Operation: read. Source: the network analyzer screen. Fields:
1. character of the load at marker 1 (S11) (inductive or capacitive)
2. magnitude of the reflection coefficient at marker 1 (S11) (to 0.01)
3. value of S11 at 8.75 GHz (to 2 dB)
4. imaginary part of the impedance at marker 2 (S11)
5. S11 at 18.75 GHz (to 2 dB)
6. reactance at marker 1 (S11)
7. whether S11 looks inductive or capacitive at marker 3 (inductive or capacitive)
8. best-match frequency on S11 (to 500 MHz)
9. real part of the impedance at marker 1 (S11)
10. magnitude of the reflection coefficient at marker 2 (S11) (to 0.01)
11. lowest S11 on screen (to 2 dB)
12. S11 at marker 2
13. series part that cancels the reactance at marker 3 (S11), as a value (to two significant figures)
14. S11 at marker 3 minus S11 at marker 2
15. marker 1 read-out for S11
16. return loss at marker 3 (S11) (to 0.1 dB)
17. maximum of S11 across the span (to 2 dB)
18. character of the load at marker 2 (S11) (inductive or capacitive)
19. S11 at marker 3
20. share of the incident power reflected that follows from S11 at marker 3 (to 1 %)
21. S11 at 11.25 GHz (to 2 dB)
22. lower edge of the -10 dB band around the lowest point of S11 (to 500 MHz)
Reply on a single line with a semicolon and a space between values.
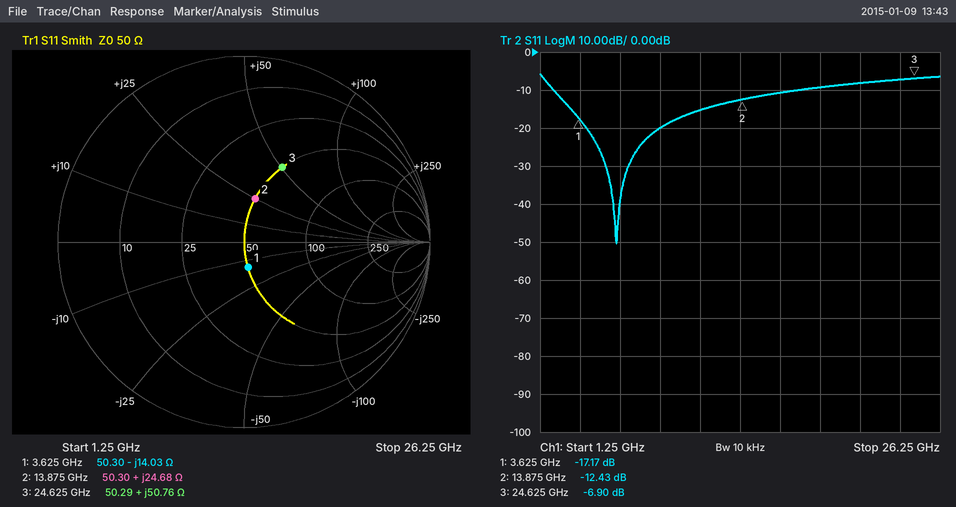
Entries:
capacitive; 0.14; -20 dB; +24.68 Ω; -10 dB; -14.03 Ω; inductive; 6.0 GHz; 50.30 Ω; 0.24; -50 dB; -12.43 dB; 130 fF; 5.53 dB; -17.17 dB; 6.9 dB; -6 dB; inductive; -6.90 dB; 20 %; -16 dB; 2.0 GHz
